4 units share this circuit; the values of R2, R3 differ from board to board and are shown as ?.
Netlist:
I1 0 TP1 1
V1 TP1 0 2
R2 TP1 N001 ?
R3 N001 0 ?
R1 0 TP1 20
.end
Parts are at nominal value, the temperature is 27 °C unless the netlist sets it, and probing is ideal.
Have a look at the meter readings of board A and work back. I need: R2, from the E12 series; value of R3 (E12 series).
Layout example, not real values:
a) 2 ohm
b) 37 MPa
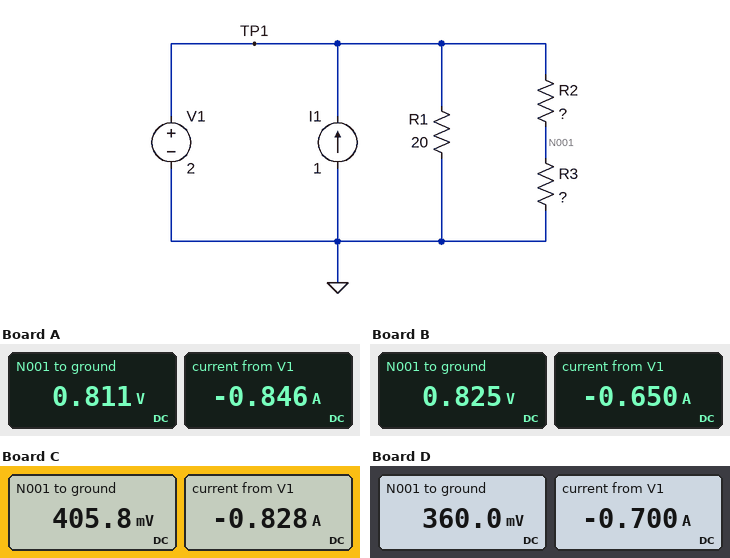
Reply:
a) 22 Ω
b) 15 Ω
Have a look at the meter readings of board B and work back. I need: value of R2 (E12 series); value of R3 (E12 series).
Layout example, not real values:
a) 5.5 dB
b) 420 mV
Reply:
a) 4.7 Ω
b) 3.3 Ω
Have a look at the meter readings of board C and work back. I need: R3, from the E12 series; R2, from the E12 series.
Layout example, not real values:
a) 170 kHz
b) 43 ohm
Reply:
a) 5.6 Ω
b) 22 Ω
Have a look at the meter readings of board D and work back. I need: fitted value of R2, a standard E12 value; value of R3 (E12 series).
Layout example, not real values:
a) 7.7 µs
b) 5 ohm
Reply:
a) 8.2 Ω
b) 1.8 Ω
